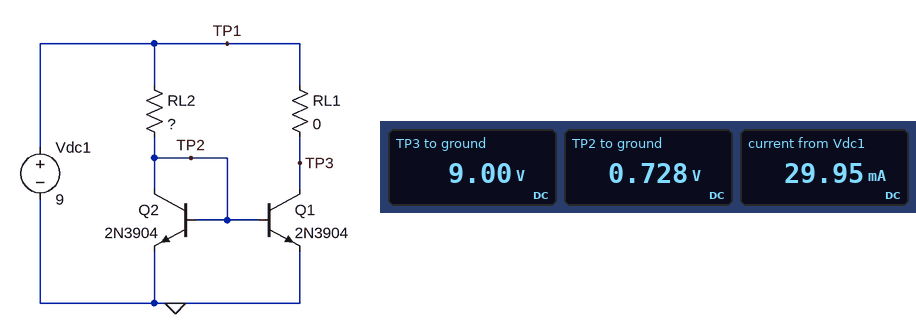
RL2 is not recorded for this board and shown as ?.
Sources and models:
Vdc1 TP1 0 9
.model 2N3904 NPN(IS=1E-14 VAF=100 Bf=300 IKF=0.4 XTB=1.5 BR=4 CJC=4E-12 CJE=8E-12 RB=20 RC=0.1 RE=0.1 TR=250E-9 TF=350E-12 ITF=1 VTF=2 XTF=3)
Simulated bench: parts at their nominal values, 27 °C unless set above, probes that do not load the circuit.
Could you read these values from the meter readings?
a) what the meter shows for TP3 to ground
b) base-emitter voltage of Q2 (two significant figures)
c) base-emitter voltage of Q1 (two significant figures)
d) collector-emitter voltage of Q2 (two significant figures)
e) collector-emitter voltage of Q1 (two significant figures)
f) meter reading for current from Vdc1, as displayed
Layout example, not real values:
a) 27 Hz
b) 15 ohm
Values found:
a) 9.00 V
b) 730 mV
c) 730 mV
d) 730 mV
e) 9.0 V
f) 29.95 mA
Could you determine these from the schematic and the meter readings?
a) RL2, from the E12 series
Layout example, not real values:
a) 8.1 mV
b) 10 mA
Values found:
a) 560 Ω
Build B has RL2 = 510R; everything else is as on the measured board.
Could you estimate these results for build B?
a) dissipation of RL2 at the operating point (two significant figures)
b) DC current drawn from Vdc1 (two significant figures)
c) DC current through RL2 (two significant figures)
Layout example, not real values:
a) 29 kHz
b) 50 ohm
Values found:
a) 130 mW
b) 34 mA
c) 16 mA
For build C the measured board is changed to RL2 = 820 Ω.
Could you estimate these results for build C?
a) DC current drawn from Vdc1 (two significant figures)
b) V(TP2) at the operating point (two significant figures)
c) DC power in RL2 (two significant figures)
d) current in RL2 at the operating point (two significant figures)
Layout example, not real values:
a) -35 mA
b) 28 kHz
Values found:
a) 23 mA
b) 720 mV
c) 84 mW
d) 10 mA
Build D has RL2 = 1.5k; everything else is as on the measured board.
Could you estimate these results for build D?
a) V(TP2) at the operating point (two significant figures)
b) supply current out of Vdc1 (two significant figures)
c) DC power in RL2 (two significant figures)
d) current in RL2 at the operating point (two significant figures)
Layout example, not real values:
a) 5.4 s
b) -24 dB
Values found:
a) 700 mV
b) 13 mA
c) 46 mW
d) 5.5 mA
